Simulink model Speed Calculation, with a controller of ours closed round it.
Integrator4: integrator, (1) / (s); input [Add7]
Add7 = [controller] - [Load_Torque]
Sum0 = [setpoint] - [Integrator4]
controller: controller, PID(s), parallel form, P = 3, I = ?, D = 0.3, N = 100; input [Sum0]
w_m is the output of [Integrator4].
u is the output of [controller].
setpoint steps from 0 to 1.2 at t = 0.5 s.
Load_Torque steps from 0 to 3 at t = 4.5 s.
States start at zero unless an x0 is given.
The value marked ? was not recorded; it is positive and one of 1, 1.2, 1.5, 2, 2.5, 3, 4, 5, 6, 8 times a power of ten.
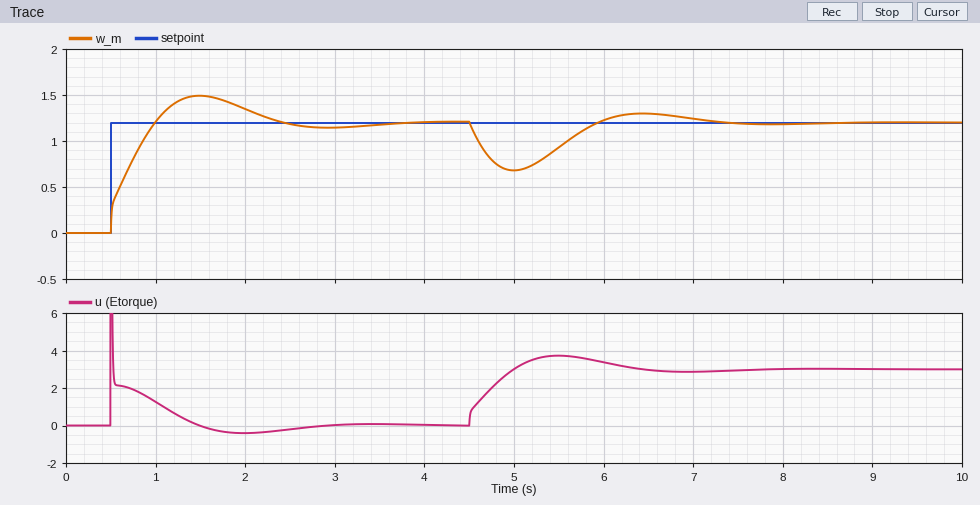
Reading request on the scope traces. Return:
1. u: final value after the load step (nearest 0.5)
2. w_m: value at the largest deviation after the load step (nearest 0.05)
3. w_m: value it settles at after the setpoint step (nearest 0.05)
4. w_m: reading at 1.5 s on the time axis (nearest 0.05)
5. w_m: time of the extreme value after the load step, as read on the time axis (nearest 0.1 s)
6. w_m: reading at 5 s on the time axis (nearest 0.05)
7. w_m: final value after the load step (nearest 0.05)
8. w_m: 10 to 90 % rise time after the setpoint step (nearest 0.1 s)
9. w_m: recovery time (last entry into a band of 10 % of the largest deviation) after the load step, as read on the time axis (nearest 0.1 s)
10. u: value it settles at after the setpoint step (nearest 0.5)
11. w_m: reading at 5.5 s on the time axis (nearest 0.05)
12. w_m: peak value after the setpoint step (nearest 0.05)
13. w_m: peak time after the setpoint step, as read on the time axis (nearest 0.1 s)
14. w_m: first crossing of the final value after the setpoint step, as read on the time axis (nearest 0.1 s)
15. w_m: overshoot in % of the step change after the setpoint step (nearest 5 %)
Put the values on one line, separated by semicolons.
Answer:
3.0; 0.70; 1.20; 1.50; 5.0 s; 0.70; 1.20; 0.4 s; 6.9 s; 0.0; 0.95; 1.50; 1.5 s; 1.0 s; 25 %
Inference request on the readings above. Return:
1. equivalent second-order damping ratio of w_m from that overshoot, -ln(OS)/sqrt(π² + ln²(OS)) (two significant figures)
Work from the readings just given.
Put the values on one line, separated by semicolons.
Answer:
0.40
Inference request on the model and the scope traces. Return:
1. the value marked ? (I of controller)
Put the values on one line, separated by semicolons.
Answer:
8
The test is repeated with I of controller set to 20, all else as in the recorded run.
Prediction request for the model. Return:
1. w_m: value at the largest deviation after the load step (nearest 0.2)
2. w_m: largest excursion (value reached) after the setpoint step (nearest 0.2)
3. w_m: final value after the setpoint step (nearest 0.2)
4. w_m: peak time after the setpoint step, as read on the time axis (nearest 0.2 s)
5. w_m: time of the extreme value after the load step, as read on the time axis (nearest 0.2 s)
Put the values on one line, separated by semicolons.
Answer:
0.8; 1.6; 1.2; 1.2 s; 4.8 s
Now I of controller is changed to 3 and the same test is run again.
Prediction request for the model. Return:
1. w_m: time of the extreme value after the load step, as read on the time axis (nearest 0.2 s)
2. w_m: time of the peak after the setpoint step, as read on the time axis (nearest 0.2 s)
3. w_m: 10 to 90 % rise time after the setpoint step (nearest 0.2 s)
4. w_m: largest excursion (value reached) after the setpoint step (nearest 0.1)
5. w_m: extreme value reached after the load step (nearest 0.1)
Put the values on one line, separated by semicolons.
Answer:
5.2 s; 2.0 s; 0.6 s; 1.4; 0.5
